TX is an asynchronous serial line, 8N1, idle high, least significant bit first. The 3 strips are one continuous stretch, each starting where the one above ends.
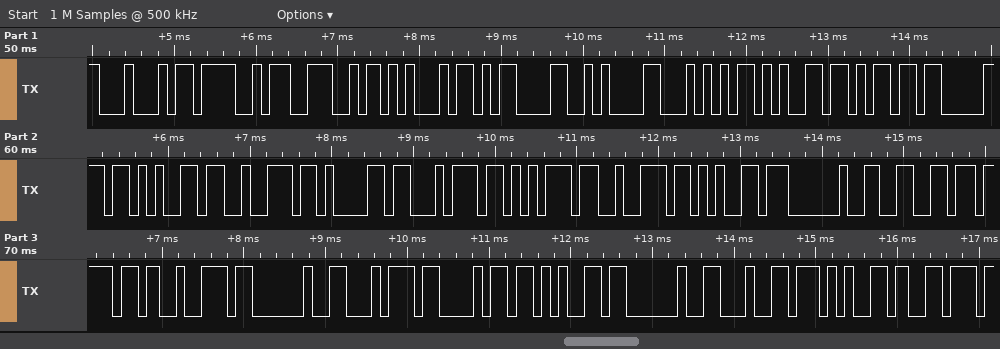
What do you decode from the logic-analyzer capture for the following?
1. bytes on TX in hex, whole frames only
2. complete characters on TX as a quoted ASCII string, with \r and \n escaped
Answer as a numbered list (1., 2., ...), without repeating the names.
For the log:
1. 44 4F 4E 45 0D 0A 54 65 6D 70 65 72 61 74 75 72 65 20 66 6F 72 20 74 68 65 20 64 65 76
2. "DONE\r\nTemperature for the dev"
